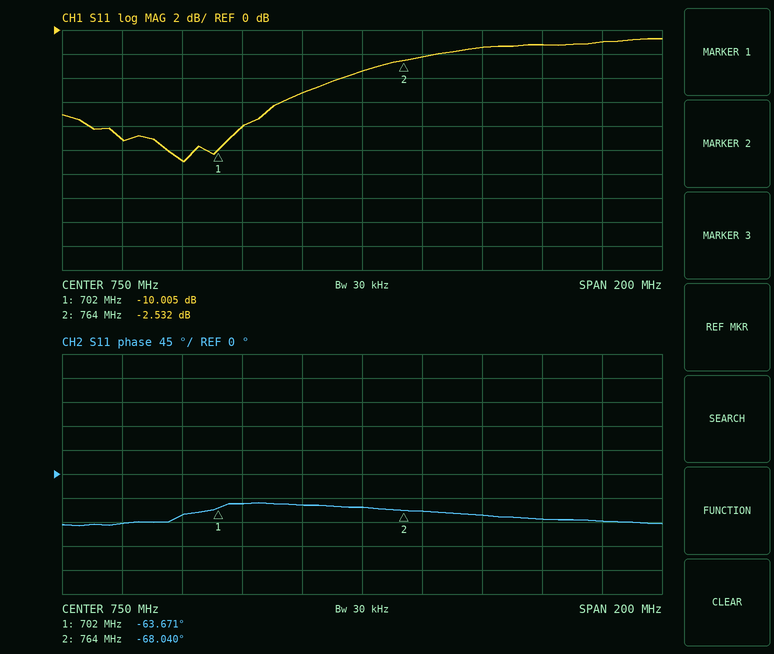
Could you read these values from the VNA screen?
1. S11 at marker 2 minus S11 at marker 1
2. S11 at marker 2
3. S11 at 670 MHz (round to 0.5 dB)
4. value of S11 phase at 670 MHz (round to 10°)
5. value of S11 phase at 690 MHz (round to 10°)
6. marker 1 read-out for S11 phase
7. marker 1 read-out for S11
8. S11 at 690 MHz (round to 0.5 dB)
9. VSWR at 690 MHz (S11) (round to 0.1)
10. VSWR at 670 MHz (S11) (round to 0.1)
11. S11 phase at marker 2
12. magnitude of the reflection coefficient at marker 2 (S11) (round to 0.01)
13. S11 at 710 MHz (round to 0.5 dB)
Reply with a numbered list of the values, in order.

1. 7.473 dB
2. -2.532 dB
3. -9.0 dB
4. -90°
5. -80°
6. -63.671°
7. -10.005 dB
8. -11.0 dB
9. 1.8
10. 2.1
11. -68.040°
12. 0.75
13. -8.0 dB
